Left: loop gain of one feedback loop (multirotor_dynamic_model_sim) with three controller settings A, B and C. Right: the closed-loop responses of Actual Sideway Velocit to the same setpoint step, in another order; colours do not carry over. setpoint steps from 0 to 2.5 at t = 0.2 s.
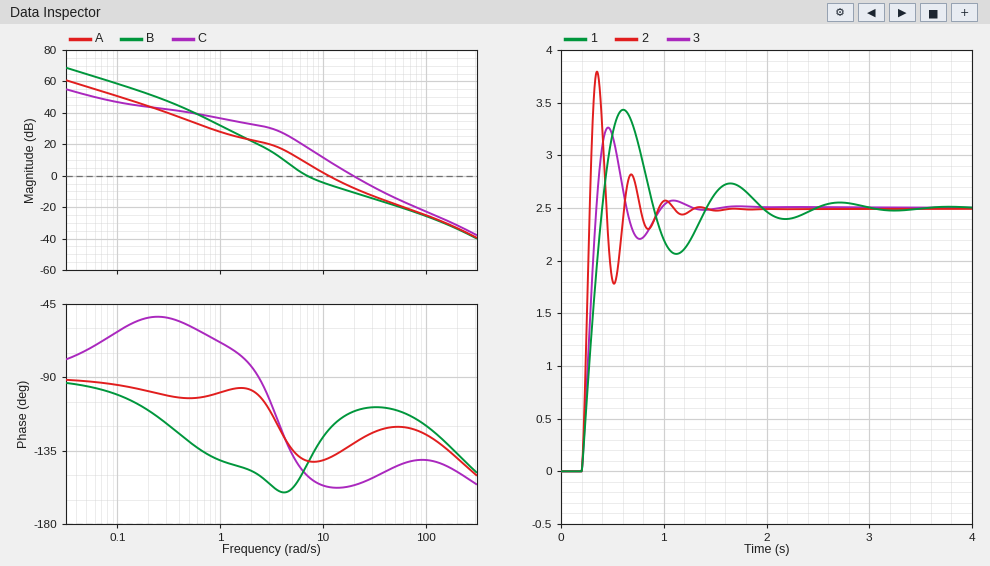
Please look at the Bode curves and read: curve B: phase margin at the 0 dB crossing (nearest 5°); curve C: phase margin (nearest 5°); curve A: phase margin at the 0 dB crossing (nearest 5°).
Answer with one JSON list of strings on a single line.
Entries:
["35°", "25°", "40°"]
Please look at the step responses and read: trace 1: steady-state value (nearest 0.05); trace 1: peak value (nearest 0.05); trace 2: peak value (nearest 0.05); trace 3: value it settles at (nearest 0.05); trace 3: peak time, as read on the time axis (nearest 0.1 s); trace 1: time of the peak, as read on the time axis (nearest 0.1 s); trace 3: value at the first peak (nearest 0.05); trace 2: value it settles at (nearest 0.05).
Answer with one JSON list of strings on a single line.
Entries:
["2.50", "3.45", "3.80", "2.50", "0.5 s", "0.6 s", "3.25", "2.50"]
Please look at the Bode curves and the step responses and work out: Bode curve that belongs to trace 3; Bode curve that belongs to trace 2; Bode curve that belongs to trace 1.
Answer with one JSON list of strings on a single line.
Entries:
["A", "C", "B"]
